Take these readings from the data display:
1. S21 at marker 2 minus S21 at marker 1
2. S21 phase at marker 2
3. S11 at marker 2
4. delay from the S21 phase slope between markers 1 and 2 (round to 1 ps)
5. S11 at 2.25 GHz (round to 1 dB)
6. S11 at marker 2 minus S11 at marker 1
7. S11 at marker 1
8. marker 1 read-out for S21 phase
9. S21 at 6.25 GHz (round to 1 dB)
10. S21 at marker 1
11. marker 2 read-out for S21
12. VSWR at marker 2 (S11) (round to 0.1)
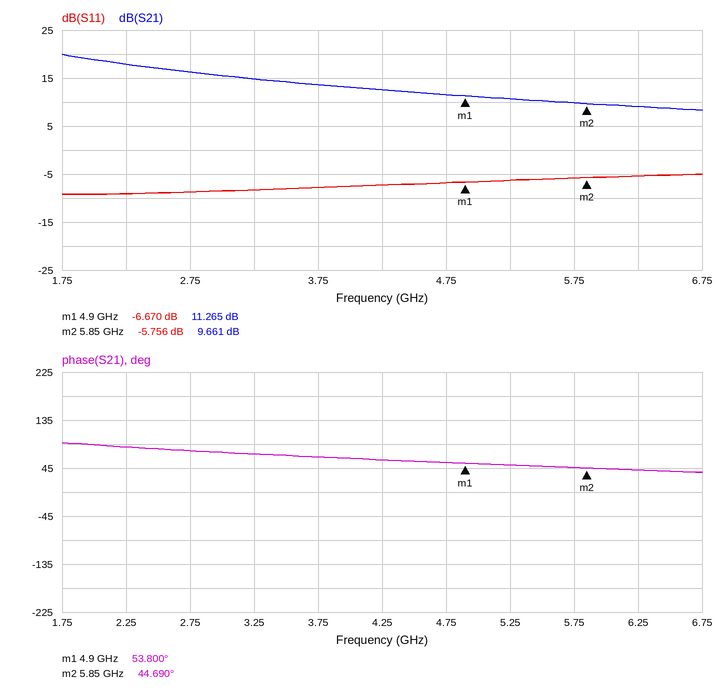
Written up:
-1.604 dB
44.690°
-5.756 dB
27 ps
-9 dB
0.914 dB
-6.670 dB
53.800°
9 dB
11.265 dB
9.661 dB
3.1
